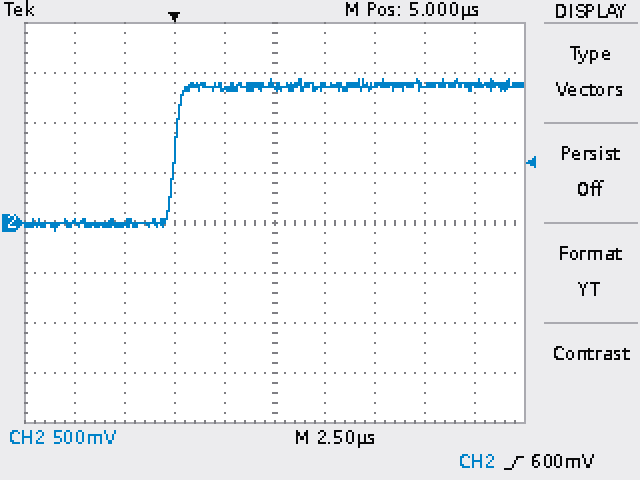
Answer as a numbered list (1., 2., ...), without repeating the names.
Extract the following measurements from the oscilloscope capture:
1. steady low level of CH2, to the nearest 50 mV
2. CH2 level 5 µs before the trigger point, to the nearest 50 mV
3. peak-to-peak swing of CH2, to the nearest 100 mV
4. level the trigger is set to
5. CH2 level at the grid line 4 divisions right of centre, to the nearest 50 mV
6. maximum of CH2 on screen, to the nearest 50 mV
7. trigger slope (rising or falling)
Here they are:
1. 0 mV
2. 0 mV
3. 1.50 V
4. 600 mV
5. 1.35 V
6. 1.45 V
7. rising
